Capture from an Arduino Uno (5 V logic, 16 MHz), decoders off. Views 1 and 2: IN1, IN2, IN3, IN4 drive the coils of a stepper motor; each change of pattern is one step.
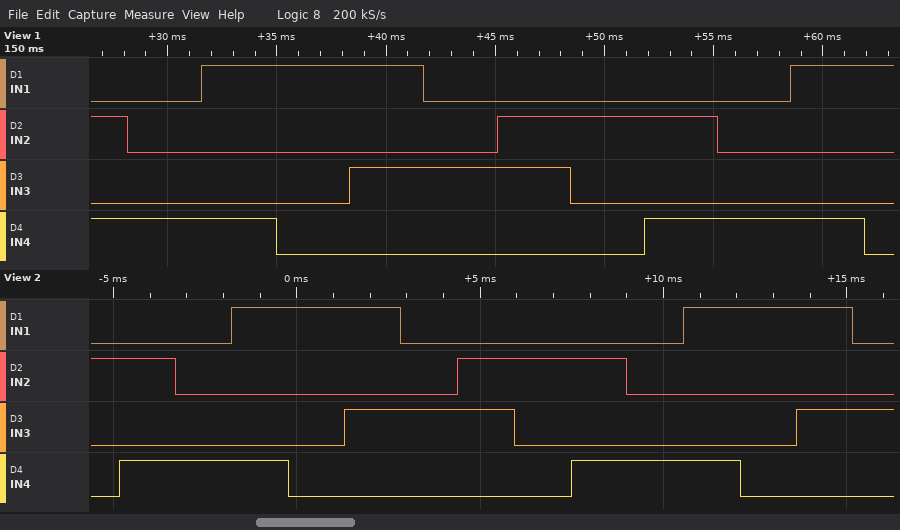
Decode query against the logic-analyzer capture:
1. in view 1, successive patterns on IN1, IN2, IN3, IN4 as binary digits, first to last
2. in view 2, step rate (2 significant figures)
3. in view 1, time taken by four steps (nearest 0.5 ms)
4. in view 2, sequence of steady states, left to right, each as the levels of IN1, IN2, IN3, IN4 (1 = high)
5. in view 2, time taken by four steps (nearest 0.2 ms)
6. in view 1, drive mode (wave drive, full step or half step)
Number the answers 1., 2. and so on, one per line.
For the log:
1. 0101 0001 1001 1000 1010 0010 0110 0100 0101 0001 1001 1000
2. 650 steps/s
3. 13.5 ms
4. 0100 0101 0001 1001 1000 1010 0010 0110 0100 0101 0001 1001 1000 1010 0010
5. 6.2 ms
6. half step
